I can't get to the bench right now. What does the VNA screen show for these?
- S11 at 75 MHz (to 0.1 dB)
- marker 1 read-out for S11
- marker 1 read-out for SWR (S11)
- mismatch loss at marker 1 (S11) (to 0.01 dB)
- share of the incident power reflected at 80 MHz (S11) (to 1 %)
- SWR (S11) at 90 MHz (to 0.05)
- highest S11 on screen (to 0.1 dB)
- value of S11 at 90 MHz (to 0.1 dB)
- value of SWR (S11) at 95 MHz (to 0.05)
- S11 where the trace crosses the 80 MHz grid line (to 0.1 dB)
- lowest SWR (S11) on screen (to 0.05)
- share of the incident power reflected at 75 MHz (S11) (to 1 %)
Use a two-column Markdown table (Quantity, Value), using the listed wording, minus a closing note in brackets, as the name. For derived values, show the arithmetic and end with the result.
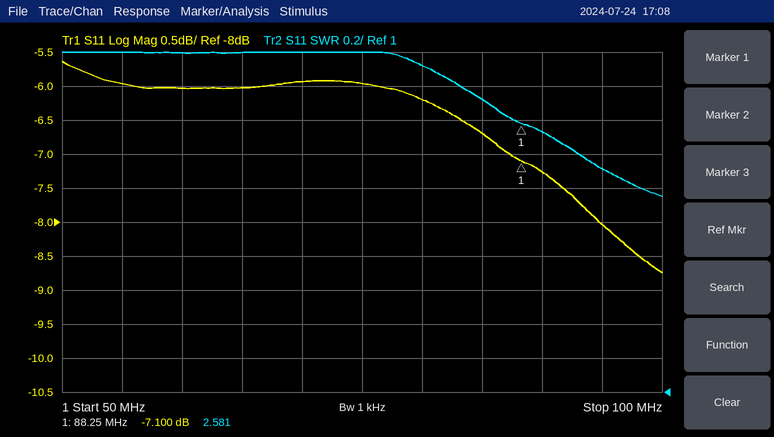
| Quantity | Value |
|---|---|
| S11 at 75 MHz | -6.0 dB |
| marker 1 read-out for S11 | -7.100 dB |
| marker 1 read-out for SWR | 2.581 |
| mismatch loss at marker 1 (S11) | −10 log10(1 − 10^(-7.1/10)) ≈ 0.94 dB |
| share of the incident power reflected at 80 MHz (S11) | 10^(-6.2/10) ≈ 24 % |
| SWR (S11) at 90 MHz | 2.55 |
| highest S11 on screen | -5.6 dB |
| value of S11 at 90 MHz | -7.3 dB |
| value of SWR (S11) at 95 MHz | 2.30 |
| S11 where the trace crosses the 80 MHz grid line | -6.2 dB |
| lowest SWR (S11) on screen | 2.15 |
| share of the incident power reflected at 75 MHz (S11) | 10^(-6/10) ≈ 25 % |
